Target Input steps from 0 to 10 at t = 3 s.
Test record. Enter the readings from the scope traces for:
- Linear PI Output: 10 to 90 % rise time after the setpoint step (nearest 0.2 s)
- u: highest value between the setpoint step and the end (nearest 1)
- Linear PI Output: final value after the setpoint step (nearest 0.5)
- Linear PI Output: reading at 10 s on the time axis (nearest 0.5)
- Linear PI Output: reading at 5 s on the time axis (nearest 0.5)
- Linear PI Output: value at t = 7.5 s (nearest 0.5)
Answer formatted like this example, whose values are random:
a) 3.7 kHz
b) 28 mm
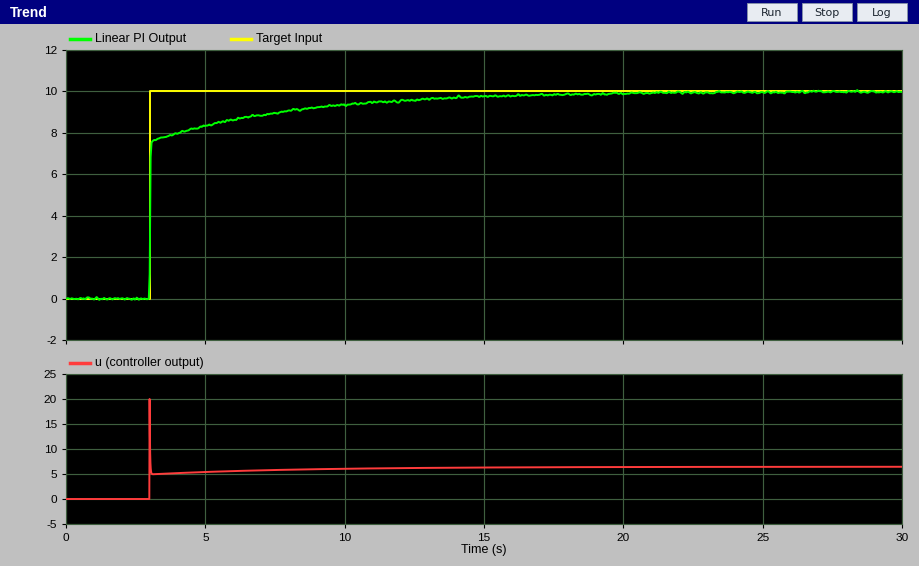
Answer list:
a) 4.6 s
b) 20
c) 10.0
d) 9.5
e) 8.5
f) 9.0
